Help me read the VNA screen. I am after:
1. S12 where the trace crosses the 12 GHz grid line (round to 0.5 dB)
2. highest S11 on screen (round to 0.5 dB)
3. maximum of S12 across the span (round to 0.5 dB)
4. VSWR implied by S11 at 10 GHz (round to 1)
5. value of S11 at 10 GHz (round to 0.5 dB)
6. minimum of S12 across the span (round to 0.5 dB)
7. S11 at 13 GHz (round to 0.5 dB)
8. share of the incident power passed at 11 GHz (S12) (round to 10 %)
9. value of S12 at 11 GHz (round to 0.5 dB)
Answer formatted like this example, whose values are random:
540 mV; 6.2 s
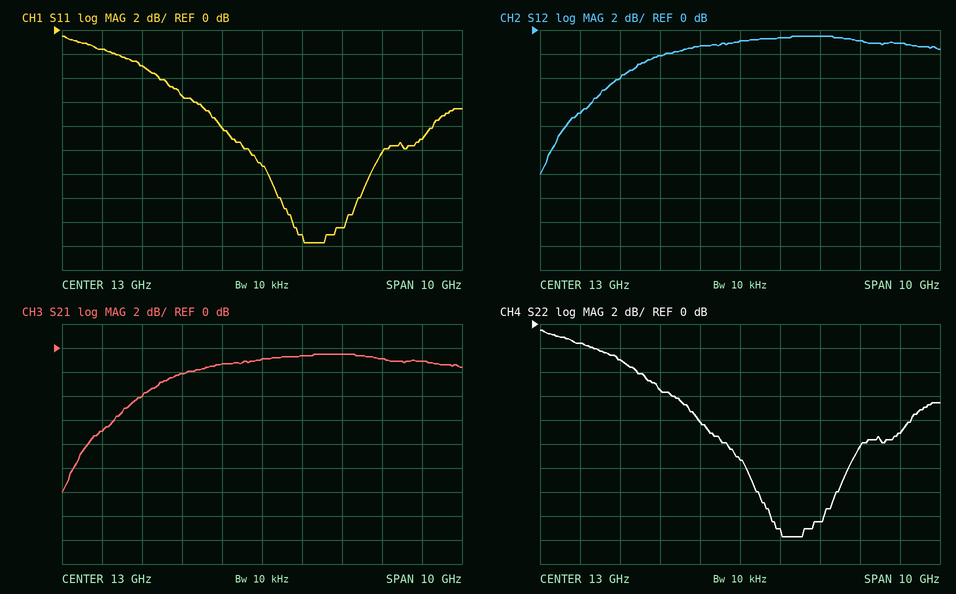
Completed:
-1.5 dB; -0.5 dB; -0.5 dB; 6; -3.0 dB; -12.0 dB; -11.5 dB; 60 %; -2.0 dB
